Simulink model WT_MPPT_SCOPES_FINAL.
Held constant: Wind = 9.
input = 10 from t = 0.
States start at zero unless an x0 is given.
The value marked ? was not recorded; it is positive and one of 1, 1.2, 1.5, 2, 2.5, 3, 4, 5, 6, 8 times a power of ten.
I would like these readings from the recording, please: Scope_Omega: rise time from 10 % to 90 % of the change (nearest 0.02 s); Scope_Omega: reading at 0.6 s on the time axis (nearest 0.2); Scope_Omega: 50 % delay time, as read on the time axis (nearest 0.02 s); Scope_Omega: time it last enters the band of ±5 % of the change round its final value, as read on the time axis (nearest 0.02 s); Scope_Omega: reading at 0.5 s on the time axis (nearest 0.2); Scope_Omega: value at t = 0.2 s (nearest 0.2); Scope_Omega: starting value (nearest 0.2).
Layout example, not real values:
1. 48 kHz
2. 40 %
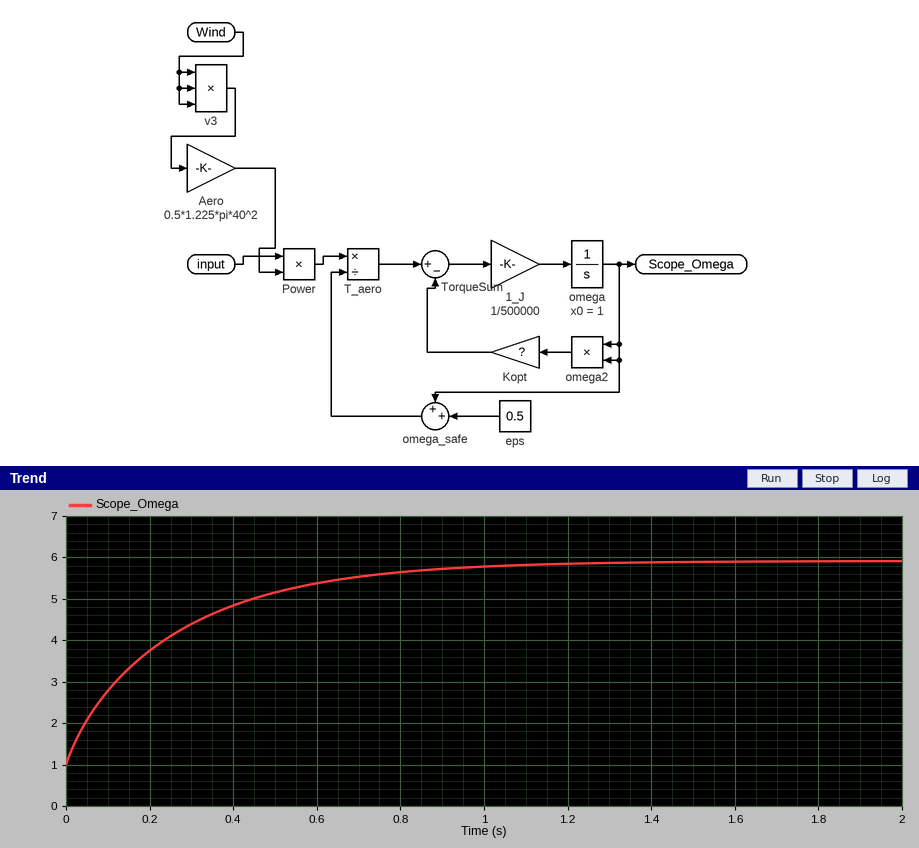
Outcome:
1. 0.60 s
2. 5.4
3. 0.16 s
4. 0.82 s
5. 5.2
6. 3.8
7. 1.0
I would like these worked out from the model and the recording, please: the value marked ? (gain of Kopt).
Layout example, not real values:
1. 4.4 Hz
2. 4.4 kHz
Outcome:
1. 100000
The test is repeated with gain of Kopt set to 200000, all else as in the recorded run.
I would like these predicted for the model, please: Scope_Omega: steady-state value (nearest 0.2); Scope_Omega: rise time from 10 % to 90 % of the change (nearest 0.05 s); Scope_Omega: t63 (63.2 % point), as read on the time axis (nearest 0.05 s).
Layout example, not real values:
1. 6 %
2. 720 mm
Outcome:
1. 4.6
2. 0.40 s
3. 0.15 s
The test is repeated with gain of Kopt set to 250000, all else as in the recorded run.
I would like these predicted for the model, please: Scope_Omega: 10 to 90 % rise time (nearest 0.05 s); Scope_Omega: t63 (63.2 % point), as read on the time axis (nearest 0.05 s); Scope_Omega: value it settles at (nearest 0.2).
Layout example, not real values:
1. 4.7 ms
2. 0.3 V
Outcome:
1. 0.35 s
2. 0.15 s
3. 4.4
